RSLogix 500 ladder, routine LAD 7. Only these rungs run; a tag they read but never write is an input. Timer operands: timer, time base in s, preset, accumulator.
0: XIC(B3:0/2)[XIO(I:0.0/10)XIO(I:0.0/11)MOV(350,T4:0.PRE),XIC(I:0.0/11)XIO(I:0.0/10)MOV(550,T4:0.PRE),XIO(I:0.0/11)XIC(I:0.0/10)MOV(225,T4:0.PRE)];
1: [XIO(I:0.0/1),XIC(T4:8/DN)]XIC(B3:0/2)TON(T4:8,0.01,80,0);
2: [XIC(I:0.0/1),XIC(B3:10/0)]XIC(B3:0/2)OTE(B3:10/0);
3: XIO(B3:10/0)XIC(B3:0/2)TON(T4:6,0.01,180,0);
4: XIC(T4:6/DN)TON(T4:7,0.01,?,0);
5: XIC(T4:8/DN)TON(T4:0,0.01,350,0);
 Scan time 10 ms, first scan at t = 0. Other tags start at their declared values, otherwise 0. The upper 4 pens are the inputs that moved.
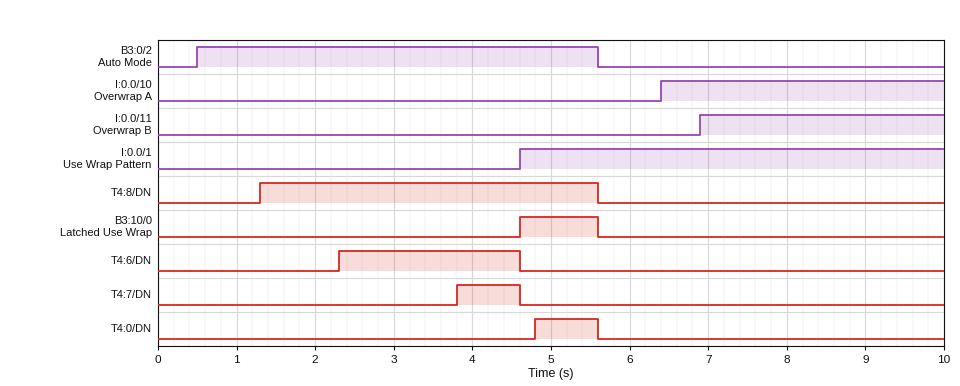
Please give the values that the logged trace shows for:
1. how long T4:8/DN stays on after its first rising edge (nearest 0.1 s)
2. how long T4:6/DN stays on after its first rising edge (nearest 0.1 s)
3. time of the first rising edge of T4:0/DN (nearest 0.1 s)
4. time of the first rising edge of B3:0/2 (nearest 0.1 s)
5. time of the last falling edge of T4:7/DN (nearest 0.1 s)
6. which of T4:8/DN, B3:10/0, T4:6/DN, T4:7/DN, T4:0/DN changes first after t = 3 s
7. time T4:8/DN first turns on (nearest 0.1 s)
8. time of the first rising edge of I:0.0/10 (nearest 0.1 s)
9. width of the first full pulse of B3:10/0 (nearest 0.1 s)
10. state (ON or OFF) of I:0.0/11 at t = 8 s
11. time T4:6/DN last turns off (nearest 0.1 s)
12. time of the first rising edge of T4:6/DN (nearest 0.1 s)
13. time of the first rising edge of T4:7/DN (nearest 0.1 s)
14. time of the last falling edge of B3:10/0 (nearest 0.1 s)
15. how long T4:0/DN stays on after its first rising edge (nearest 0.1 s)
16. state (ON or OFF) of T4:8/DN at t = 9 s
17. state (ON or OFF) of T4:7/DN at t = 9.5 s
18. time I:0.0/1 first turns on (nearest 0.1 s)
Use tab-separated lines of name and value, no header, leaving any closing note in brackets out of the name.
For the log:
how long T4:8/DN stays on after its first rising edge	4.3 s
how long T4:6/DN stays on after its first rising edge	2.3 s
time of the first rising edge of T4:0/DN	4.8 s
time of the first rising edge of B3:0/2	0.5 s
time of the last falling edge of T4:7/DN	4.6 s
which of T4:8/DN, B3:10/0, T4:6/DN, T4:7/DN, T4:0/DN changes first after t = 3 s	T4:7/DN
time T4:8/DN first turns on	1.3 s
time of the first rising edge of I:0.0/10	6.4 s
width of the first full pulse of B3:10/0	1.0 s
state (ON or OFF) of I:0.0/11 at t = 8 s	ON
time T4:6/DN last turns off	4.6 s
time of the first rising edge of T4:6/DN	2.3 s
time of the first rising edge of T4:7/DN	3.8 s
time of the last falling edge of B3:10/0	5.6 s
how long T4:0/DN stays on after its first rising edge	0.8 s
state (ON or OFF) of T4:8/DN at t = 9 s	OFF
state (ON or OFF) of T4:7/DN at t = 9.5 s	OFF
time I:0.0/1 first turns on	4.6 s
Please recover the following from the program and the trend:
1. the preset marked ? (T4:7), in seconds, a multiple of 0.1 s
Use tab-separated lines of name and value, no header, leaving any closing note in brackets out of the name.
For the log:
the preset marked ? (T4:7), in seconds, a multiple of 0.1 s	1.5 s
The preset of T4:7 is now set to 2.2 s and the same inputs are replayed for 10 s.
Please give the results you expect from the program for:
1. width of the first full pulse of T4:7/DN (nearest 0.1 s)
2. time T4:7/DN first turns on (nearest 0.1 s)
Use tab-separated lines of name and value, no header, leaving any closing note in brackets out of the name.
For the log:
width of the first full pulse of T4:7/DN	0.1 s
time T4:7/DN first turns on	4.5 s
